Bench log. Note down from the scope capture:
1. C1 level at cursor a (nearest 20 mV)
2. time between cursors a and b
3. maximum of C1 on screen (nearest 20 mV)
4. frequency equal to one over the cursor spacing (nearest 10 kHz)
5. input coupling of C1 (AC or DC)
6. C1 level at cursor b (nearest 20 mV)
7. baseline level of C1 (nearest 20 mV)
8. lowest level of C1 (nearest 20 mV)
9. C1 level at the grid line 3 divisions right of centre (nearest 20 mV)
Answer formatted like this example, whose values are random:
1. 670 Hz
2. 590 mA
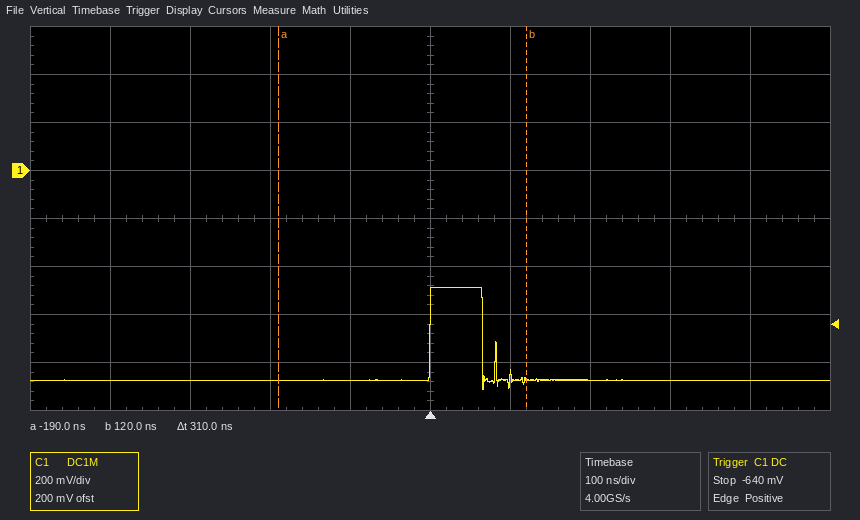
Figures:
1. -880 mV
2. 310 ns
3. -480 mV
4. 3.23 MHz
5. DC
6. -880 mV
7. -880 mV
8. -920 mV
9. -880 mV
